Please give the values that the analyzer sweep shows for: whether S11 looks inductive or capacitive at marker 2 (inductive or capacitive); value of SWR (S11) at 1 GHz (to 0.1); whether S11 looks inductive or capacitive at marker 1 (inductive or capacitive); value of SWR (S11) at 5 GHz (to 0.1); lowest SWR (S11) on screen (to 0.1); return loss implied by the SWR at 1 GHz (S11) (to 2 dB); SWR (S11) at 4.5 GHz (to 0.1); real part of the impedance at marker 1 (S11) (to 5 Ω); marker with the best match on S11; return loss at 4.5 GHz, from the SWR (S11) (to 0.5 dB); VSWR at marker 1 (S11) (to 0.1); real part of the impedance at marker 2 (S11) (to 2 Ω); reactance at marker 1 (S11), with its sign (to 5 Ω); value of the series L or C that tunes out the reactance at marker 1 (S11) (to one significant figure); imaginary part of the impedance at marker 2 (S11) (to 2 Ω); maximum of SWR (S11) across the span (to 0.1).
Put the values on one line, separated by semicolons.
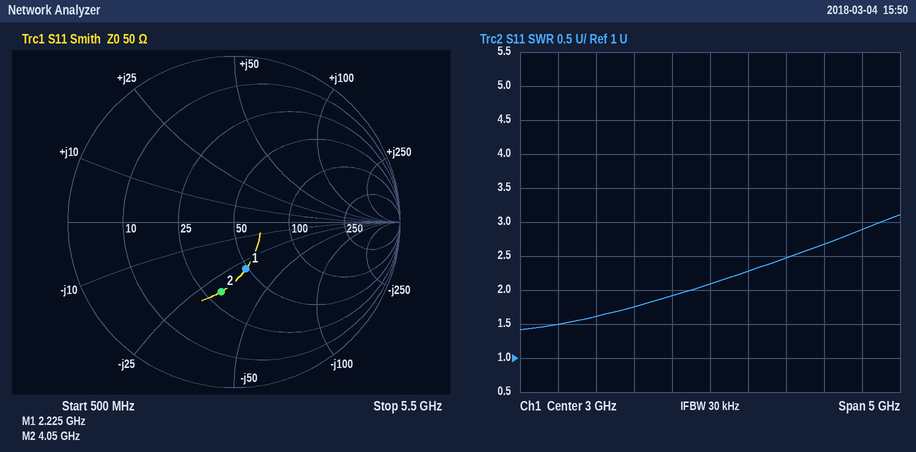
capacitive; 1.5; capacitive; 2.9; 1.4; 14 dB; 2.7; 50 Ω; marker 1; 7.0 dB; 1.8; 30 Ω; -30 Ω; 2 nH; -32 Ω; 3.1
